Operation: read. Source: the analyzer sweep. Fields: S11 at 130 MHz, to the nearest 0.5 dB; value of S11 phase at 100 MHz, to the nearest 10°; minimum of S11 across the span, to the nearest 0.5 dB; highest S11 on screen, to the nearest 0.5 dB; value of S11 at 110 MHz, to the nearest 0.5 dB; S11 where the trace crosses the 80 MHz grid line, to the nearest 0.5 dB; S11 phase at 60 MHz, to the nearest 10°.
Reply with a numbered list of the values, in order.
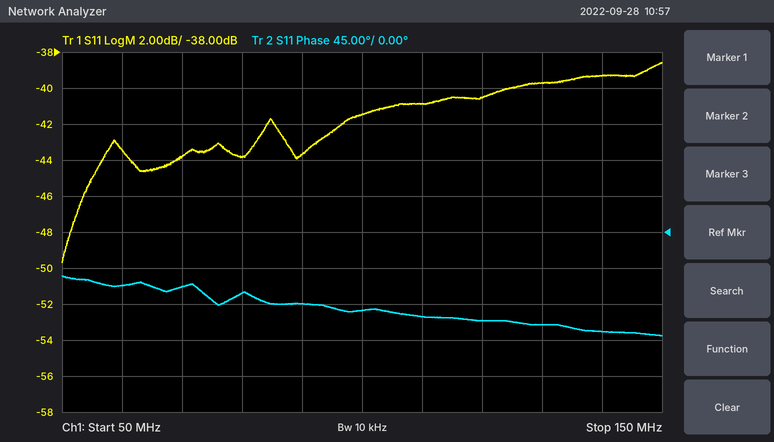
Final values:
1. -39.5 dB
2. -100°
3. -49.5 dB
4. -38.5 dB
5. -41.0 dB
6. -44.0 dB
7. -70°
